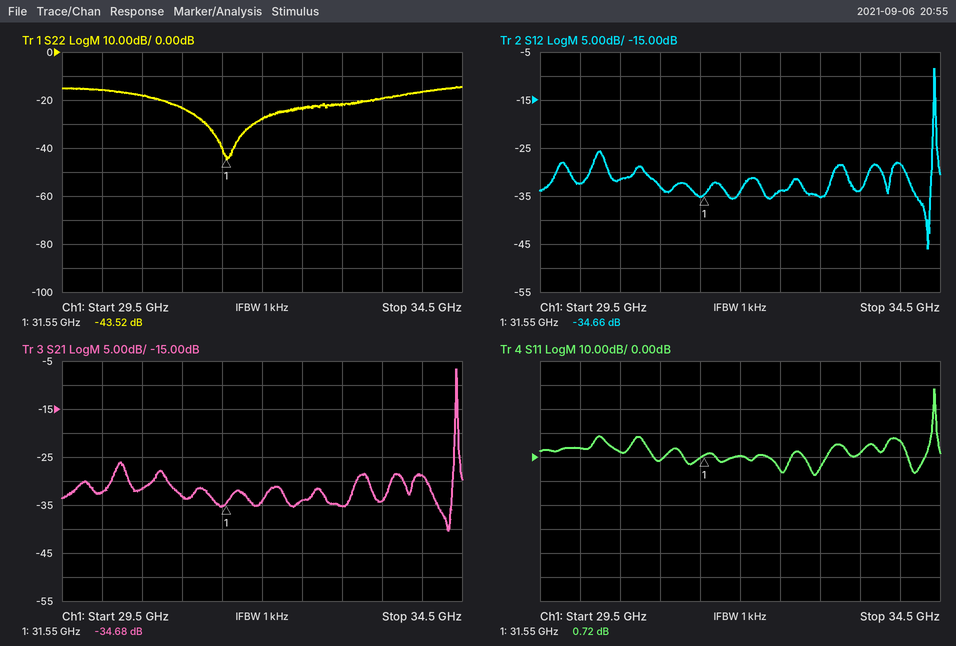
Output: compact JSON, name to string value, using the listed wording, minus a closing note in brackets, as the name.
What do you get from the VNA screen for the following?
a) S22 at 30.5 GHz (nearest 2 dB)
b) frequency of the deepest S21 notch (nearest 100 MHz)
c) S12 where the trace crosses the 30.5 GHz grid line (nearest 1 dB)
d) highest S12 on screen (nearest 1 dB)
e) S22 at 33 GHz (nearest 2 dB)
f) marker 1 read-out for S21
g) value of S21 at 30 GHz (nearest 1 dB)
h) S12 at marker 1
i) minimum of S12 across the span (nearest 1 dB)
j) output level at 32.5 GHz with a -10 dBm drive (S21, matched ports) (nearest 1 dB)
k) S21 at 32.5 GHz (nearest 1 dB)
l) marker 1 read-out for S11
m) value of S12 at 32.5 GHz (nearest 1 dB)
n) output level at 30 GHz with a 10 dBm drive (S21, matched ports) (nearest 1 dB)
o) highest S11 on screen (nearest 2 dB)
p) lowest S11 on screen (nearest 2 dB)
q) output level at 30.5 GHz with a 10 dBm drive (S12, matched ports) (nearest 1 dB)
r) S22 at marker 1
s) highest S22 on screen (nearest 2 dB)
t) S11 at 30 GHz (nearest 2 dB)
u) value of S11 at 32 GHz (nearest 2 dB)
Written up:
{"S22 at 30.5 GHz": "-18 dB", "frequency of the deepest S21 notch": "34.3 GHz", "S12 where the trace crosses the 30.5 GHz grid line": "-32 dB", "highest S12 on screen": "-8 dB", "S22 at 33 GHz": "-22 dB", "marker 1 read-out for S21": "-34.68 dB", "value of S21 at 30 GHz": "-32 dB", "S12 at marker 1": "-34.66 dB", "minimum of S12 across the span": "-46 dB", "output level at 32.5 GHz with a -10 dBm drive (S21, matched ports)": "-44 dBm", "S21 at 32.5 GHz": "-34 dB", "marker 1 read-out for S11": "0.72 dB", "value of S12 at 32.5 GHz": "-34 dB", "output level at 30 GHz with a 10 dBm drive (S21, matched ports)": "-22 dBm", "highest S11 on screen": "28 dB", "lowest S11 on screen": "-8 dB", "output level at 30.5 GHz with a 10 dBm drive (S12, matched ports)": "-22 dBm", "S22 at marker 1": "-43.52 dB", "highest S22 on screen": "-14 dB", "S11 at 30 GHz": "4 dB", "value of S11 at 32 GHz": "0 dB"}
